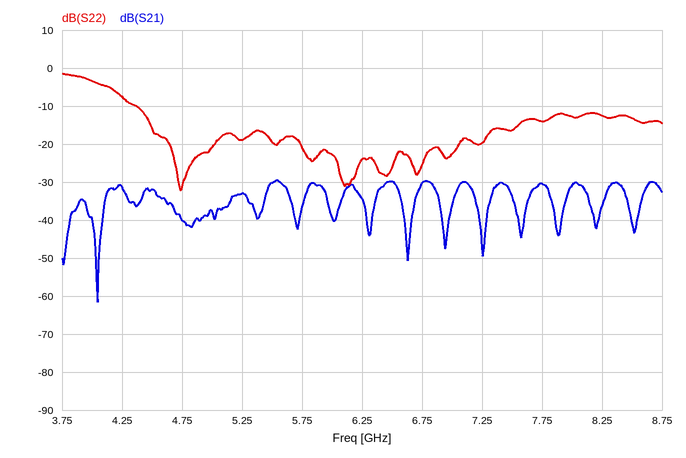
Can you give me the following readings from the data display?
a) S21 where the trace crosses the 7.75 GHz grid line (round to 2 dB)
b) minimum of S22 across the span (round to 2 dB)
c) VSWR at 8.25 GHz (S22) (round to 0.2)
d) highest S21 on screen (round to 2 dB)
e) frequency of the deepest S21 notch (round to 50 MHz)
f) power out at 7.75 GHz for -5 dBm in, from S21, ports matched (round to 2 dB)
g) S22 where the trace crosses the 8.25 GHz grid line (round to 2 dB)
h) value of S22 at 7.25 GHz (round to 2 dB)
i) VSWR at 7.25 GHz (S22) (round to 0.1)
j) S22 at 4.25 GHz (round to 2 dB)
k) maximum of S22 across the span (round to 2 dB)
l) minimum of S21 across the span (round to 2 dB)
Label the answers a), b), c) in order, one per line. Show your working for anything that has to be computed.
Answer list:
a) -30 dB
b) -32 dB
c) |Γ| = 10^(-12/20) = 0.2512; VSWR = (1 + 0.2512)/(1 − 0.2512) ≈ 1.67, so 1.6 to the nearest 0.2
d) -30 dB
e) 4.05 GHz
f) -5 dBm + (-30 dB) = -36 dBm
g) -12 dB
h) -20 dB
i) |Γ| = 10^(-20/20) = 0.1000; VSWR = (1 + 0.1000)/(1 − 0.1000) ≈ 1.2
j) -8 dB
k) -2 dB
l) -62 dB
